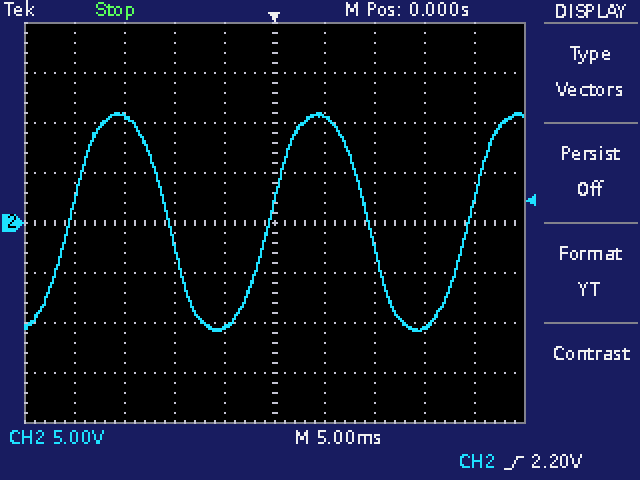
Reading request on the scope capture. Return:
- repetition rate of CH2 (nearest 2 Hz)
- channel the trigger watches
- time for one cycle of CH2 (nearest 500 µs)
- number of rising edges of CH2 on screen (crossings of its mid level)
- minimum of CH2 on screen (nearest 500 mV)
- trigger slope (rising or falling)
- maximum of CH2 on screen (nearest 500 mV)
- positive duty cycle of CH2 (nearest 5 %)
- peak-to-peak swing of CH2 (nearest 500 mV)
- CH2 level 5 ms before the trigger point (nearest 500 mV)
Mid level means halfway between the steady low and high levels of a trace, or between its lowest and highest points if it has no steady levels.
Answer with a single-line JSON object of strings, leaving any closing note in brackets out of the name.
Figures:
{"repetition rate of CH2": "50 Hz", "channel the trigger watches": "CH2", "time for one cycle of CH2": "20.0 ms", "number of rising edges of CH2 on screen": "3", "minimum of CH2 on screen": "-11.0 V", "trigger slope": "rising", "maximum of CH2 on screen": "11.0 V", "positive duty cycle of CH2": "50 %", "peak-to-peak swing of CH2": "22.0 V", "CH2 level 5 ms before the trigger point": "-10.5 V"}
